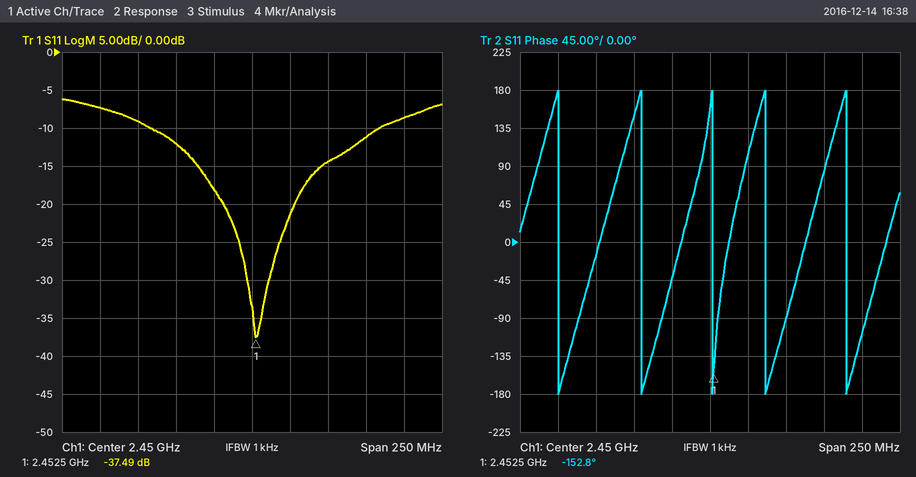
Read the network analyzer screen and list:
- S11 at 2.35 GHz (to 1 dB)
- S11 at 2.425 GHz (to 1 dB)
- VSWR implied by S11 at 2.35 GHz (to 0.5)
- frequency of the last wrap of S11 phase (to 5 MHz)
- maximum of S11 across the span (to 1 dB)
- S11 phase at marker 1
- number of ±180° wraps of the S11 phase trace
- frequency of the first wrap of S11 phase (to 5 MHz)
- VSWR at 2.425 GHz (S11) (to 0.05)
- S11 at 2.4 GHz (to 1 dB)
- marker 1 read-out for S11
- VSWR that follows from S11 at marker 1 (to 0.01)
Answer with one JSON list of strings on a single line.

["-7 dB", "-18 dB", "2.5", "2.540 GHz", "-6 dB", "-152.8°", "5", "2.350 GHz", "1.30", "-12 dB", "-37.49 dB", "1.03"]
